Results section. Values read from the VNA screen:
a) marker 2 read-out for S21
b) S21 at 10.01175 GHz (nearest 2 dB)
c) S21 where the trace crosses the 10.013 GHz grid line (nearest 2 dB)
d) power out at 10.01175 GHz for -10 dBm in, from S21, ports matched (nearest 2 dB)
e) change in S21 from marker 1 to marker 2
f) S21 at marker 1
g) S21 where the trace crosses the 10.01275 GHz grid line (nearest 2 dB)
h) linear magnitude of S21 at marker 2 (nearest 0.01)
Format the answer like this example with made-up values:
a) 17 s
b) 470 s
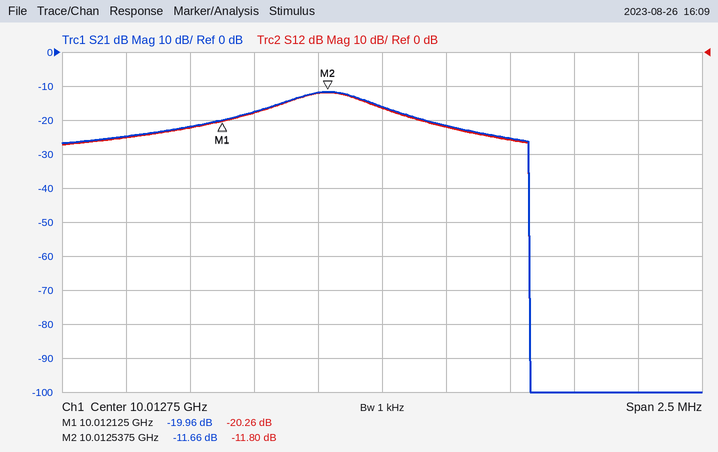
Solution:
a) -11.66 dB
b) -24 dB
c) -22 dB
d) -34 dBm
e) 8.30 dB
f) -19.96 dB
g) -16 dB
h) 0.26
